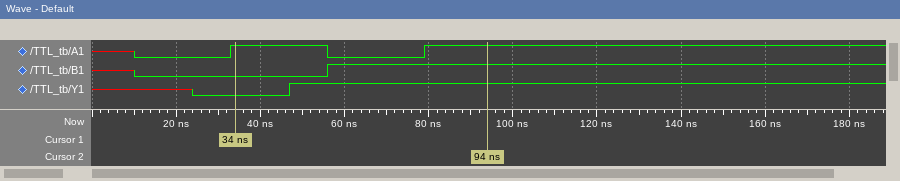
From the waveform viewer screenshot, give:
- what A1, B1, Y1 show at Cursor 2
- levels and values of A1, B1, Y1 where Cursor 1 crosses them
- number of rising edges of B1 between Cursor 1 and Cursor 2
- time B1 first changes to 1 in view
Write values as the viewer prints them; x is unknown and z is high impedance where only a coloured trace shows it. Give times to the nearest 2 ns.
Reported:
A1=1, B1=1, Y1=1
A1=1, B1=0, Y1=0
1
56 ns
